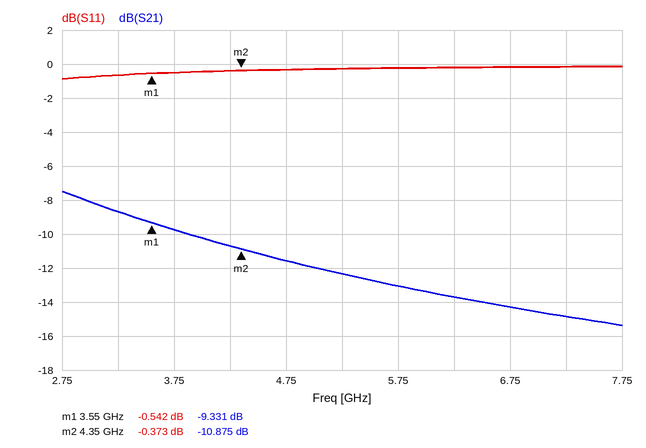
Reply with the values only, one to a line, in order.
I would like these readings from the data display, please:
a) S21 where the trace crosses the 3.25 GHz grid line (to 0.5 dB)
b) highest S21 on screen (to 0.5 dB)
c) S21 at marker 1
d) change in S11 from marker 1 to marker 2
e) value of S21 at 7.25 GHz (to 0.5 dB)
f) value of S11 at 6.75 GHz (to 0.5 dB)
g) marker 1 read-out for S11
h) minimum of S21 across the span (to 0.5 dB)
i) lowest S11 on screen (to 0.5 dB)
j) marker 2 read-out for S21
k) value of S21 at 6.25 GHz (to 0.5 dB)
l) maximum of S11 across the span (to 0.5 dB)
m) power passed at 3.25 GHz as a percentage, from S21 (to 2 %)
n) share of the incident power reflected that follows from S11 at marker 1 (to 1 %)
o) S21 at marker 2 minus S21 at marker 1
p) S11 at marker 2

-8.5 dB
-7.5 dB
-9.331 dB
0.169 dB
-15.0 dB
0.0 dB
-0.542 dB
-15.5 dB
-1.0 dB
-10.875 dB
-13.5 dB
0.0 dB
14 %
88 %
-1.544 dB
-0.373 dB
